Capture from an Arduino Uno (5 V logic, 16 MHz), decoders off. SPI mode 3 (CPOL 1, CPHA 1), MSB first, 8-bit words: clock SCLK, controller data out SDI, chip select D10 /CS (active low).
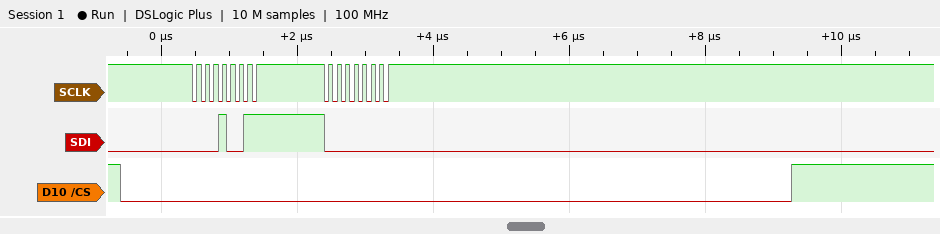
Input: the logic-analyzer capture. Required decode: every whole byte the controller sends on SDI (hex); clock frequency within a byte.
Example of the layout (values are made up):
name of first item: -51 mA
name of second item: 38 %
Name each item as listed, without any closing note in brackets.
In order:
every whole byte the controller sends on SDI: 13 00
clock frequency within a byte: 8 MHz
